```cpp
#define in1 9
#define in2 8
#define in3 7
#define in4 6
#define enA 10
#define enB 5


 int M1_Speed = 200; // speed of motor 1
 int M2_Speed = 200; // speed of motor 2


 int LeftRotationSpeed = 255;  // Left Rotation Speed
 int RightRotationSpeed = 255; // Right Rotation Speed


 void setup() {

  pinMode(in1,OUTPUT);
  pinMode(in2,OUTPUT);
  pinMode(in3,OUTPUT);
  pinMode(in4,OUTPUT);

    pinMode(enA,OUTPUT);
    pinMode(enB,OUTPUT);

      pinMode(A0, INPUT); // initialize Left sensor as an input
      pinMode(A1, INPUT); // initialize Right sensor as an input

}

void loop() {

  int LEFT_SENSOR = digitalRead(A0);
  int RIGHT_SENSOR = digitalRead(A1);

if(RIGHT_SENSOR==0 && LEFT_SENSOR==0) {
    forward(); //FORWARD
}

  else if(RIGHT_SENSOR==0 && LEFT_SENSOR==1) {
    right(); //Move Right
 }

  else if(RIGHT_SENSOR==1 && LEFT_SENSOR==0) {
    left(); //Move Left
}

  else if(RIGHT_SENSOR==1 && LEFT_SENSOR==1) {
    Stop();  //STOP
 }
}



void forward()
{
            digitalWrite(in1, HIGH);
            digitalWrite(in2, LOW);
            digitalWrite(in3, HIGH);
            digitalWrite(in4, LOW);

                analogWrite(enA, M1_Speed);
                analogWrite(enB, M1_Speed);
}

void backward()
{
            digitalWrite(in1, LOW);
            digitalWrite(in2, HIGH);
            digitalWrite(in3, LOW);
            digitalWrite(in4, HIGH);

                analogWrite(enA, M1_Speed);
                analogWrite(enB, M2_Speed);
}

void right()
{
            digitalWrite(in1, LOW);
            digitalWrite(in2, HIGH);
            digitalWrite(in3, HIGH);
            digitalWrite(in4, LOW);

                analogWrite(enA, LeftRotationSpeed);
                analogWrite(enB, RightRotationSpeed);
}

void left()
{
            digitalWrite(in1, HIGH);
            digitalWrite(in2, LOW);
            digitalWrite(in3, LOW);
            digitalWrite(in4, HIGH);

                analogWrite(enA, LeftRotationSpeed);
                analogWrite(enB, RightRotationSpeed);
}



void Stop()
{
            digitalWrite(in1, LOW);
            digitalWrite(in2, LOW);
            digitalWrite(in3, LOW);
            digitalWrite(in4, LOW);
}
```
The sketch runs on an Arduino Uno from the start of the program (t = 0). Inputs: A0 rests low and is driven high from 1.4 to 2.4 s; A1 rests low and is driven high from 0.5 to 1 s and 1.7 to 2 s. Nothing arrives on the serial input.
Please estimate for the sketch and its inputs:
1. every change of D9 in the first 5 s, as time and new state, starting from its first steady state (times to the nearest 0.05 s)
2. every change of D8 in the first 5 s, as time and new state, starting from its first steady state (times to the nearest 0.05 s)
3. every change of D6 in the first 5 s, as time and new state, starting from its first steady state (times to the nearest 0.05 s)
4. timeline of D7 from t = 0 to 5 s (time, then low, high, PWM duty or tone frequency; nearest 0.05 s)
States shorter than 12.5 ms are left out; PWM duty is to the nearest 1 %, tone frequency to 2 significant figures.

0 s high; 1.4 s low; 2.4 s high
0 s low; 1.4 s high; 1.7 s low; 2 s high; 2.4 s low
0 s low; 0.5 s high; 1 s low
0 s high; 0.5 s low; 1 s high; 1.7 s low; 2 s high
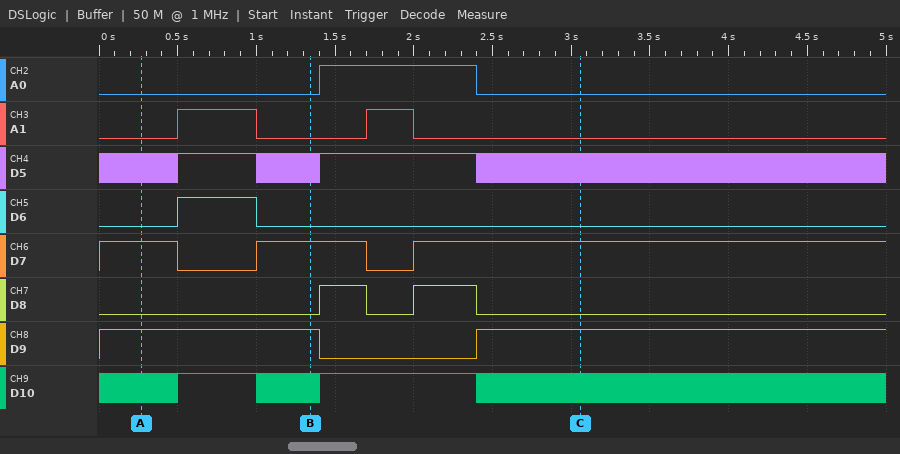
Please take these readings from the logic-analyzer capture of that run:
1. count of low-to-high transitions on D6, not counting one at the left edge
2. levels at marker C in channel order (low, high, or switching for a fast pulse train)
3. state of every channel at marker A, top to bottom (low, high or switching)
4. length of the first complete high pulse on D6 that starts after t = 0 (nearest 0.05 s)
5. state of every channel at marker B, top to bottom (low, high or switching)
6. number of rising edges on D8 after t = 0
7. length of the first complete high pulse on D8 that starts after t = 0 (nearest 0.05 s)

1
A0 low, A1 low, D5 switching, D6 low, D7 high, D8 low, D9 high, D10 switching
A0 low, A1 low, D5 switching, D6 low, D7 high, D8 low, D9 high, D10 switching
0.50 s
A0 low, A1 low, D5 switching, D6 low, D7 high, D8 low, D9 high, D10 switching
2
0.30 s
